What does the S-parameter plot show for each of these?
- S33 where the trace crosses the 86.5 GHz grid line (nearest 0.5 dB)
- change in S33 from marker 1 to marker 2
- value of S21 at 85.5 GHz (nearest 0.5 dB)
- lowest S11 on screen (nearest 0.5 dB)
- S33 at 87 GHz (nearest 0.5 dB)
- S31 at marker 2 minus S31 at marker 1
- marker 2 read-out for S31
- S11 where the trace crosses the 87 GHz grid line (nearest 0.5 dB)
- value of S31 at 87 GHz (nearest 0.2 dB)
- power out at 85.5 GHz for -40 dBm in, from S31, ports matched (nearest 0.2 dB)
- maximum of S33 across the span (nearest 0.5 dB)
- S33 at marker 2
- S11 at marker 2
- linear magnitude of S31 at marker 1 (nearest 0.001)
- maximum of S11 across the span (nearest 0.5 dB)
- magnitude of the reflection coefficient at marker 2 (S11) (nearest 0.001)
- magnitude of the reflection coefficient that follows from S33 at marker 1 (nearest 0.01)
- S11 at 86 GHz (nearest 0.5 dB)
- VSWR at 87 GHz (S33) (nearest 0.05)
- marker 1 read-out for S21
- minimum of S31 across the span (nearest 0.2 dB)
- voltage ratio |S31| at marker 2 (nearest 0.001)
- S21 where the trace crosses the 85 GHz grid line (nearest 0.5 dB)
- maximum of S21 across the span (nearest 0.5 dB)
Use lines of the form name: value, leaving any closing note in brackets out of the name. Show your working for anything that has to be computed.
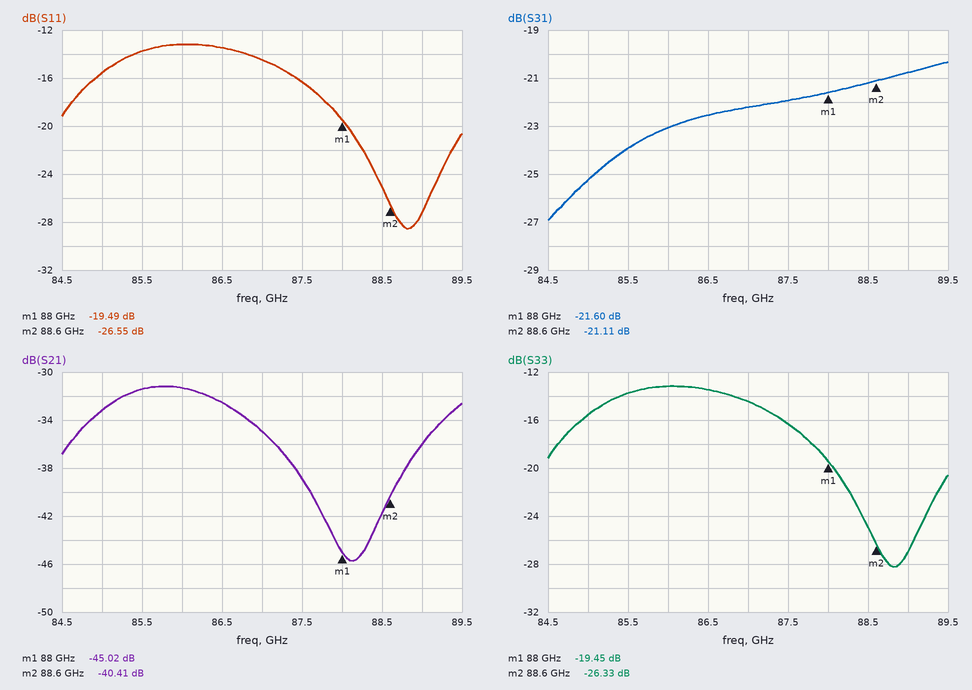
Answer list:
S33 where the trace crosses the 86.5 GHz grid line: -13.5 dB
change in S33 from marker 1 to marker 2: -26.33 − (-19.45) = -6.88 dB
value of S21 at 85.5 GHz: -31.5 dB
lowest S11 on screen: -28.5 dB
S33 at 87 GHz: -14.5 dB
S31 at marker 2 minus S31 at marker 1: -21.11 − (-21.6) = 0.49 dB
marker 2 read-out for S31: -21.11 dB
S11 where the trace crosses the 87 GHz grid line: -14.5 dB
value of S31 at 87 GHz: -22.2 dB
power out at 85.5 GHz for -40 dBm in, from S31, ports matched: -40 dBm + (-24.0 dB) = -64.0 dBm
maximum of S33 across the span: -13.0 dB
S33 at marker 2: -26.33 dB
S11 at marker 2: -26.55 dB
linear magnitude of S31 at marker 1: 10^(-21.6/20) ≈ 0.083
maximum of S11 across the span: -13.0 dB
magnitude of the reflection coefficient at marker 2 (S11): 10^(-26.55/20) ≈ 0.047
magnitude of the reflection coefficient that follows from S33 at marker 1: 10^(-19.45/20) ≈ 0.11
S11 at 86 GHz: -13.0 dB
VSWR at 87 GHz (S33): |Γ| = 10^(-14.5/20) = 0.1884; VSWR = (1 + 0.1884)/(1 − 0.1884) ≈ 1.46, so 1.45 to the nearest 0.05
marker 1 read-out for S21: -45.02 dB
minimum of S31 across the span: -27.0 dB
voltage ratio |S31| at marker 2: 10^(-21.11/20) ≈ 0.088
S21 where the trace crosses the 85 GHz grid line: -33.0 dB
maximum of S21 across the span: -31.0 dB
